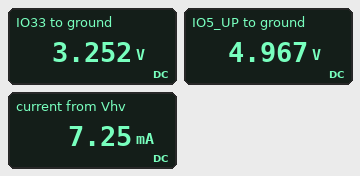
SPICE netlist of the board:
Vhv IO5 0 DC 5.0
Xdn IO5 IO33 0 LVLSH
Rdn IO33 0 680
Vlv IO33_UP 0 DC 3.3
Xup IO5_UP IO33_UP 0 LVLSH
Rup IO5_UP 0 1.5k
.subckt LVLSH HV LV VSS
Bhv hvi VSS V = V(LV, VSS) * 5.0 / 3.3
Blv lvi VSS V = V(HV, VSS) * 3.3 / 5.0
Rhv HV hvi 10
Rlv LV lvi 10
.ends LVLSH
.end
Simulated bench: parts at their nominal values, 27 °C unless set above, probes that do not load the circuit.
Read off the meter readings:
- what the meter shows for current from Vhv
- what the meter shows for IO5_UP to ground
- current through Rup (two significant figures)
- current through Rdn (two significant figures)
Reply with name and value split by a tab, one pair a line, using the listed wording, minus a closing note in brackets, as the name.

what the meter shows for current from Vhv	7.25 mA
what the meter shows for IO5_UP to ground	4.967 V
current through Rup	3.3 mA
current through Rdn	4.8 mA
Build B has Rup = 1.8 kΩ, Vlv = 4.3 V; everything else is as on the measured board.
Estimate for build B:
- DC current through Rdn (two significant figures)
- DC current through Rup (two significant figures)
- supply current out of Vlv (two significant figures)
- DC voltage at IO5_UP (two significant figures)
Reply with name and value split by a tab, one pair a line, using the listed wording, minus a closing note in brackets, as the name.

DC current through Rdn	4.8 mA
DC current through Rup	3.6 mA
supply current out of Vlv	2.4 mA
DC voltage at IO5_UP	6.5 V
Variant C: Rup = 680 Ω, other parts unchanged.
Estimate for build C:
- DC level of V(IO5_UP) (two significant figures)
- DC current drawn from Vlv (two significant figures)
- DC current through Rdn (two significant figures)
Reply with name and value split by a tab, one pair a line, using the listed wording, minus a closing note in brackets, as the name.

DC level of V(IO5_UP)	4.9 V
DC current drawn from Vlv	4.8 mA
DC current through Rdn	4.8 mA
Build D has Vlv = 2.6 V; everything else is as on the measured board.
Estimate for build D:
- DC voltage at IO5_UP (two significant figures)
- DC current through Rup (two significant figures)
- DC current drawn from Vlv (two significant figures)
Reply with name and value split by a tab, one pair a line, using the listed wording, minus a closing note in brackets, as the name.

DC voltage at IO5_UP	3.9 V
DC current through Rup	2.6 mA
DC current drawn from Vlv	1.7 mA
